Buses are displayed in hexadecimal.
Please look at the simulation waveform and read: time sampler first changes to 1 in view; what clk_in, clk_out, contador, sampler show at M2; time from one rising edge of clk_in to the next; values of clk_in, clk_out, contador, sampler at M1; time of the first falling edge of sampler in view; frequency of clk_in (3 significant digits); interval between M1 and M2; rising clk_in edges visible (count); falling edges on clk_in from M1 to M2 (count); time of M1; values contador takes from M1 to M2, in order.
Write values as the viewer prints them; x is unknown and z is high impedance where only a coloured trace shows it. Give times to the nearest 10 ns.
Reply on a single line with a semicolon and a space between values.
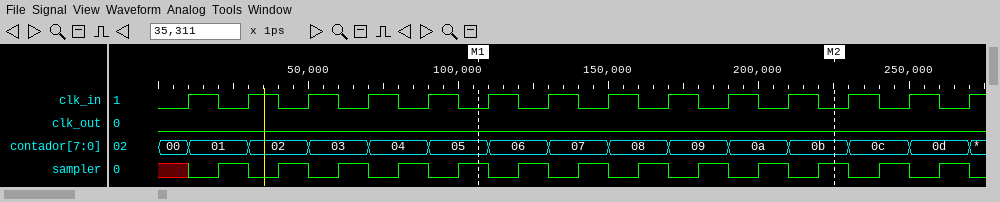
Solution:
20 ns; clk_in=0, clk_out=0, contador=0b, sampler=1; 20 ns; clk_in=0, clk_out=0, contador=05, sampler=1; 30 ns; 50.0 MHz; 120 ns; 14; 6; 110 ns; 05, 06, 07, 08, 09, 0a, 0b
